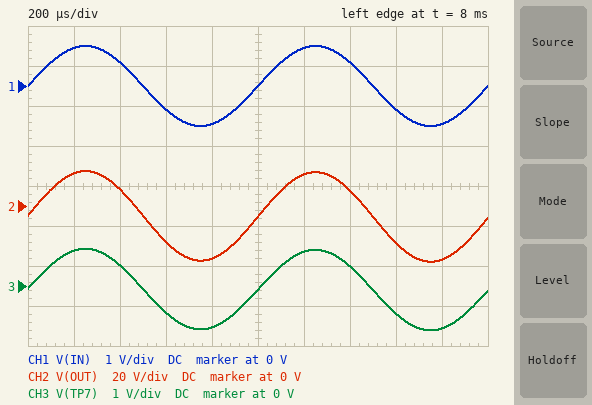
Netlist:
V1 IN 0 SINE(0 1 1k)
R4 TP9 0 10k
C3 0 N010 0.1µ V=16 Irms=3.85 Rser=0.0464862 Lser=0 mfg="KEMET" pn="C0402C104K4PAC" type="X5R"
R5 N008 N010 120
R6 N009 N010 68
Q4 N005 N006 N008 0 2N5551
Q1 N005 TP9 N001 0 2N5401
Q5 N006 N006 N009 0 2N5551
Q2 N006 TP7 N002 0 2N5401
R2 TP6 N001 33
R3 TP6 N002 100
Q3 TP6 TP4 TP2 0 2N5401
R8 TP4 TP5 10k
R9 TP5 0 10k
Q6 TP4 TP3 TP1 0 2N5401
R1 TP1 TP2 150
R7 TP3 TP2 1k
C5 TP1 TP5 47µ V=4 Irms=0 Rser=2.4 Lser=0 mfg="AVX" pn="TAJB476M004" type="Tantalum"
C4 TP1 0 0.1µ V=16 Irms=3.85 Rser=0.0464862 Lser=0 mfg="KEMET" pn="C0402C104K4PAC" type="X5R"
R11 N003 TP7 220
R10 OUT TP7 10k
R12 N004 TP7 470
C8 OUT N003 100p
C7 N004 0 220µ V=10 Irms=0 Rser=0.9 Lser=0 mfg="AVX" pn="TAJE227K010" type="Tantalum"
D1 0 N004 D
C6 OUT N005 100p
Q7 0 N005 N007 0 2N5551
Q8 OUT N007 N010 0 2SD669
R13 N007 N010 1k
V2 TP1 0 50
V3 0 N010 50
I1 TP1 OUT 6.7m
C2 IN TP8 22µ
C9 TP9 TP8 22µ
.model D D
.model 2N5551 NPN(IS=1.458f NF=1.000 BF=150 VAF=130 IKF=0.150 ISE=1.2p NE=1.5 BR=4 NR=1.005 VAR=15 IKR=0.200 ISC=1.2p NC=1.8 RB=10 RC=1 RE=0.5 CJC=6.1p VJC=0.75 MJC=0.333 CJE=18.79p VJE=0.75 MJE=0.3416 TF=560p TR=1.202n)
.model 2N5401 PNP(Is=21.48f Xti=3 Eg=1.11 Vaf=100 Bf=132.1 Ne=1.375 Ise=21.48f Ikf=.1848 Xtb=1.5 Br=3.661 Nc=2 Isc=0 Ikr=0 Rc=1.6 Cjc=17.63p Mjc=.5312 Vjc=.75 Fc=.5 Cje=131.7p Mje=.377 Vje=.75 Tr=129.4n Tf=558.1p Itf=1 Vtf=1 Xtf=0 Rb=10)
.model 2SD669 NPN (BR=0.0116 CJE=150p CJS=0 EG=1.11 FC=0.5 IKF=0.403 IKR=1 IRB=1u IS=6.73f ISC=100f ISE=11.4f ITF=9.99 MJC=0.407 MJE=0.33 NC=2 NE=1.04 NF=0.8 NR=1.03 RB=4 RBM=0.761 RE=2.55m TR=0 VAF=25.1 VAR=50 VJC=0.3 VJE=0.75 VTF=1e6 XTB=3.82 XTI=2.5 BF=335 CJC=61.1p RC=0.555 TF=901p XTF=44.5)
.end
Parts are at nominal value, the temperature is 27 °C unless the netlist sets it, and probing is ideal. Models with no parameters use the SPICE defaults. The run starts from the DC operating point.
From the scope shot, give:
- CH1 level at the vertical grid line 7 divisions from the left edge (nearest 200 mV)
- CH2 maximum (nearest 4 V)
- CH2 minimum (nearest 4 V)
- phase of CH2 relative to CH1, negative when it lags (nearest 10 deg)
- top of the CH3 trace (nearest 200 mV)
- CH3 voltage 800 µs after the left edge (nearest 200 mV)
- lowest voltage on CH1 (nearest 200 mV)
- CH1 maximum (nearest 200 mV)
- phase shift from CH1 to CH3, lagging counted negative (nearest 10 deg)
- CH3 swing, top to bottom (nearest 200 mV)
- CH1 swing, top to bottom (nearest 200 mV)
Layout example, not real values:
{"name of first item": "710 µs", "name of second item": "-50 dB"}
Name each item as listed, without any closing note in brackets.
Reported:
{"CH1 level at the vertical grid line 7 divisions from the left edge": "600 mV", "CH2 maximum": "16 V", "CH2 minimum": "-28 V", "phase of CH2 relative to CH1, negative when it lags": "0 deg", "top of the CH3 trace": "1.0 V", "CH3 voltage 800 µs after the left edge": "-1.0 V", "lowest voltage on CH1": "-1.0 V", "CH1 maximum": "1.0 V", "phase shift from CH1 to CH3, lagging counted negative": "0 deg", "CH3 swing, top to bottom": "2.0 V", "CH1 swing, top to bottom": "2.0 V"}
